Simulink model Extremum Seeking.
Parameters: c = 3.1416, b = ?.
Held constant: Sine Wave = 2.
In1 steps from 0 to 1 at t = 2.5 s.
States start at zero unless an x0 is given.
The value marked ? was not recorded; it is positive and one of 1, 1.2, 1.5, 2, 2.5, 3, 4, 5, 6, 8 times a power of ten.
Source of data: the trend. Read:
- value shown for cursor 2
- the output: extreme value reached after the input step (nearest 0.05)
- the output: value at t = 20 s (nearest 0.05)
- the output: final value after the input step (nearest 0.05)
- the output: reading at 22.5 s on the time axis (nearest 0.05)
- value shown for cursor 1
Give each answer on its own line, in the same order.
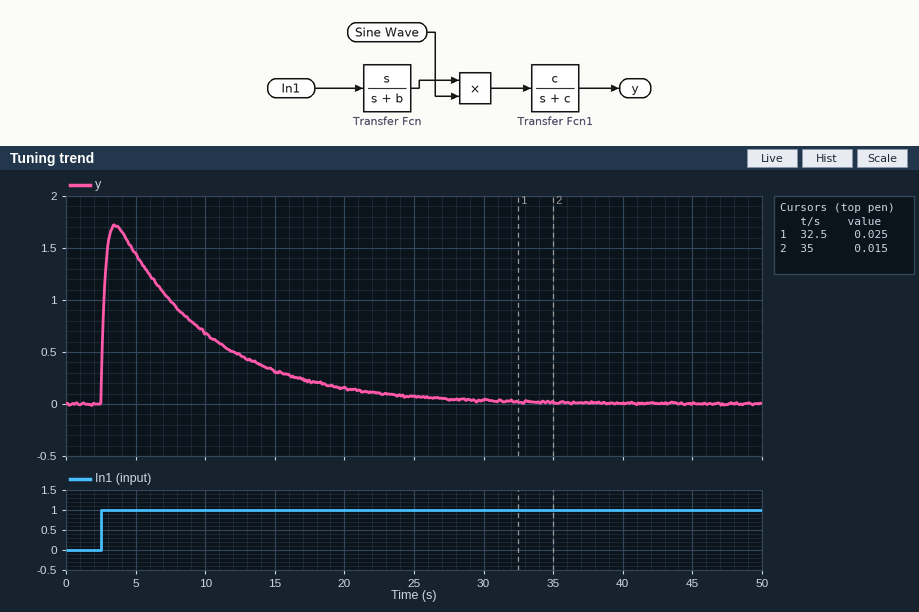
0.015
1.70
0.15
0.00
0.10
0.025
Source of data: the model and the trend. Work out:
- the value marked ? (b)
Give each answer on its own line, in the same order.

0.15
